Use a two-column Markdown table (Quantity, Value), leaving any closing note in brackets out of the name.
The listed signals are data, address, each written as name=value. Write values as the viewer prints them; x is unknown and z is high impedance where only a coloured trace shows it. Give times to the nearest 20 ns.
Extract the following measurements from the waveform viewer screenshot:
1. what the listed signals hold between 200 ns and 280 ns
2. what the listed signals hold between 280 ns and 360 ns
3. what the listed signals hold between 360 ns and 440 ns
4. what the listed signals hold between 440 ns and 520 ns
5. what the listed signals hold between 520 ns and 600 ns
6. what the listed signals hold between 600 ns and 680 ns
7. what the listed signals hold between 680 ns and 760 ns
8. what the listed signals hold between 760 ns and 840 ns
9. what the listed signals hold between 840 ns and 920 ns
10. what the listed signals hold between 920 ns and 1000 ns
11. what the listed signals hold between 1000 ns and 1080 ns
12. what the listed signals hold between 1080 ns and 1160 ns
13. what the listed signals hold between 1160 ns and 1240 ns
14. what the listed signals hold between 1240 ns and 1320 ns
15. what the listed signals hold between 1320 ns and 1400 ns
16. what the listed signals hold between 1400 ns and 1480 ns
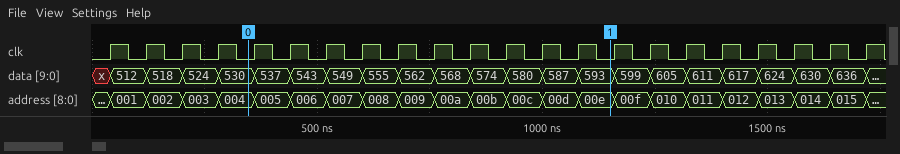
| Quantity | Value |
|---|---|
| what the listed signals hold between 200 ns and 280 ns | data=524, address=003 |
| what the listed signals hold between 280 ns and 360 ns | data=530, address=004 |
| what the listed signals hold between 360 ns and 440 ns | data=537, address=005 |
| what the listed signals hold between 440 ns and 520 ns | data=543, address=006 |
| what the listed signals hold between 520 ns and 600 ns | data=549, address=007 |
| what the listed signals hold between 600 ns and 680 ns | data=555, address=008 |
| what the listed signals hold between 680 ns and 760 ns | data=562, address=009 |
| what the listed signals hold between 760 ns and 840 ns | data=568, address=00a |
| what the listed signals hold between 840 ns and 920 ns | data=574, address=00b |
| what the listed signals hold between 920 ns and 1000 ns | data=580, address=00c |
| what the listed signals hold between 1000 ns and 1080 ns | data=587, address=00d |
| what the listed signals hold between 1080 ns and 1160 ns | data=593, address=00e |
| what the listed signals hold between 1160 ns and 1240 ns | data=599, address=00f |
| what the listed signals hold between 1240 ns and 1320 ns | data=605, address=010 |
| what the listed signals hold between 1320 ns and 1400 ns | data=611, address=011 |
| what the listed signals hold between 1400 ns and 1480 ns | data=617, address=012 |
